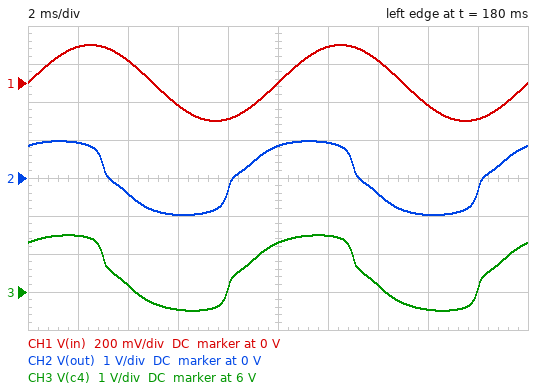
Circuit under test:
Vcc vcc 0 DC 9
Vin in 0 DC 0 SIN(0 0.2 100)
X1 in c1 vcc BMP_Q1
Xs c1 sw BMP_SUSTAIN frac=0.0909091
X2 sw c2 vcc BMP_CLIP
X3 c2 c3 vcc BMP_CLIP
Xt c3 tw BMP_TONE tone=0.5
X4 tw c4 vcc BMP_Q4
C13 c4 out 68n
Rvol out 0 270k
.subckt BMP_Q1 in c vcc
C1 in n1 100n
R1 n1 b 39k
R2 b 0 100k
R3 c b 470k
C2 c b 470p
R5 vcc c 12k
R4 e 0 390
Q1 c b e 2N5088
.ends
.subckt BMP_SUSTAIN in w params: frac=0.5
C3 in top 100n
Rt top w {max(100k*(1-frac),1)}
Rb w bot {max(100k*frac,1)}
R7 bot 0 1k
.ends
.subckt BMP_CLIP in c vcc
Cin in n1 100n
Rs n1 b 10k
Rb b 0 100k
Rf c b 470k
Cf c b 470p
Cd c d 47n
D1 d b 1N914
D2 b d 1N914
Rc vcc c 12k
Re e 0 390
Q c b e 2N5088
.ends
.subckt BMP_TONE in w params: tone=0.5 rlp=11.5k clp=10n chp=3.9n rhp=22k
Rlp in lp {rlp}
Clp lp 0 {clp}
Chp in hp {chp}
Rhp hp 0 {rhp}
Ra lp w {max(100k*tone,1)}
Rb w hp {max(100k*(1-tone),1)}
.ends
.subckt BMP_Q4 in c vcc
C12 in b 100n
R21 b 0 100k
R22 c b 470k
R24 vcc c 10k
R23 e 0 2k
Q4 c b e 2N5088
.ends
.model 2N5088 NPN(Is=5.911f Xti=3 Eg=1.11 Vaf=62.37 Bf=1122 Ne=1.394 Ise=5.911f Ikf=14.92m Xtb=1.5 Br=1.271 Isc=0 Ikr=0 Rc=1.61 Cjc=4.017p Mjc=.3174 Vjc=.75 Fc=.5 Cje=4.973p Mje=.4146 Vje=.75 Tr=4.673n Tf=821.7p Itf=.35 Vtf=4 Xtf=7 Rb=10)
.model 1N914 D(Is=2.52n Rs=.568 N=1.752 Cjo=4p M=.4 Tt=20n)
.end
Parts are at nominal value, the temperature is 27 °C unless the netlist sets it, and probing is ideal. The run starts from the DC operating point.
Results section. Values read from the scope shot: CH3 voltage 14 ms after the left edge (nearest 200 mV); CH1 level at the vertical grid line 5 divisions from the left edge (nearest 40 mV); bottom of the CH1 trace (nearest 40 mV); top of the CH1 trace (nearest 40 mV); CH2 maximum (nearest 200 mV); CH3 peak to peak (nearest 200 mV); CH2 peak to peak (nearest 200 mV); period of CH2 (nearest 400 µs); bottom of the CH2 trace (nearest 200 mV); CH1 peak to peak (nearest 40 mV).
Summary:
6.2 V
0 V
-200 mV
200 mV
1.0 V
2.0 V
2.0 V
10.0 ms
-1.0 V
400 mV
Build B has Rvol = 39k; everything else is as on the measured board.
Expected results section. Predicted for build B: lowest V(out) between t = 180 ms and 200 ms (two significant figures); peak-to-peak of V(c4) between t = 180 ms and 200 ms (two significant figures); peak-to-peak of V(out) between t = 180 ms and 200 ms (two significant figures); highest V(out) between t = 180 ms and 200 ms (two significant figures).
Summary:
-770 mV
1.8 V
1.5 V
760 mV
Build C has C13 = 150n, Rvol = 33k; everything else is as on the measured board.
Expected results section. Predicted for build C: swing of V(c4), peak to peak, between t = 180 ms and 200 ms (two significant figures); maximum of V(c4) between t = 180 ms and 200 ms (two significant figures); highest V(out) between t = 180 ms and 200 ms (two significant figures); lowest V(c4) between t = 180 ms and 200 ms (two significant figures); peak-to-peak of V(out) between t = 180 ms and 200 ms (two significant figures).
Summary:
1.7 V
7.4 V
780 mV
5.6 V
1.6 V
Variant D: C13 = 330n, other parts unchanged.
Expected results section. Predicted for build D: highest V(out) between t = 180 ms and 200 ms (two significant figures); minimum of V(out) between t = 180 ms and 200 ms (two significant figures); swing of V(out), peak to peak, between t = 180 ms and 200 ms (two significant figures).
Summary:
980 mV
-990 mV
2.0 V
